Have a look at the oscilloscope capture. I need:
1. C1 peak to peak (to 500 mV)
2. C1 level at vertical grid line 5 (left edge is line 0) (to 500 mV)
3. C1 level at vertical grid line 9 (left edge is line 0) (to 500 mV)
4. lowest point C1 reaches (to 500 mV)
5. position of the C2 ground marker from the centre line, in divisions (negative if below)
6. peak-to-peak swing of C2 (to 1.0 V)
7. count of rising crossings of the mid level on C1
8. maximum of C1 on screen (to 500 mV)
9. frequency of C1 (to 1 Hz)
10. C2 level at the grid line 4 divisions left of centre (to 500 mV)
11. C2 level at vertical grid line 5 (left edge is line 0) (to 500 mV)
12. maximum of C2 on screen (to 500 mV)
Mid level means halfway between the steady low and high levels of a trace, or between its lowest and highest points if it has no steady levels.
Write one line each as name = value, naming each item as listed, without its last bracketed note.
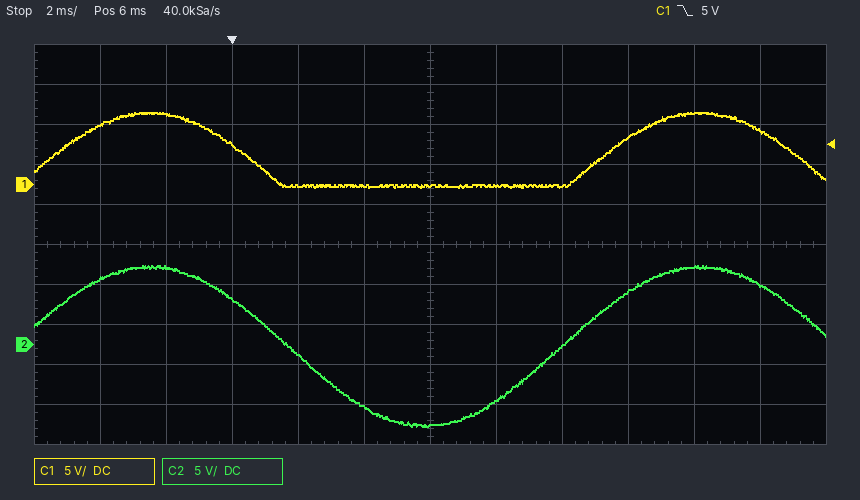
C1 peak to peak = 9.5 V
C1 level at vertical grid line 5 (left edge is line 0) = 0.0 V
C1 level at vertical grid line 9 (left edge is line 0) = 6.0 V
lowest point C1 reaches = -500 mV
position of the C2 ground marker from the centre line, in divisions = -2.5 div
peak-to-peak swing of C2 = 20.0 V
count of rising crossings of the mid level on C1 = 2
maximum of C1 on screen = 9.0 V
frequency of C1 = 60 Hz
C2 level at the grid line 4 divisions left of centre = 9.5 V
C2 level at vertical grid line 5 (left edge is line 0) = -8.0 V
maximum of C2 on screen = 10.0 V
